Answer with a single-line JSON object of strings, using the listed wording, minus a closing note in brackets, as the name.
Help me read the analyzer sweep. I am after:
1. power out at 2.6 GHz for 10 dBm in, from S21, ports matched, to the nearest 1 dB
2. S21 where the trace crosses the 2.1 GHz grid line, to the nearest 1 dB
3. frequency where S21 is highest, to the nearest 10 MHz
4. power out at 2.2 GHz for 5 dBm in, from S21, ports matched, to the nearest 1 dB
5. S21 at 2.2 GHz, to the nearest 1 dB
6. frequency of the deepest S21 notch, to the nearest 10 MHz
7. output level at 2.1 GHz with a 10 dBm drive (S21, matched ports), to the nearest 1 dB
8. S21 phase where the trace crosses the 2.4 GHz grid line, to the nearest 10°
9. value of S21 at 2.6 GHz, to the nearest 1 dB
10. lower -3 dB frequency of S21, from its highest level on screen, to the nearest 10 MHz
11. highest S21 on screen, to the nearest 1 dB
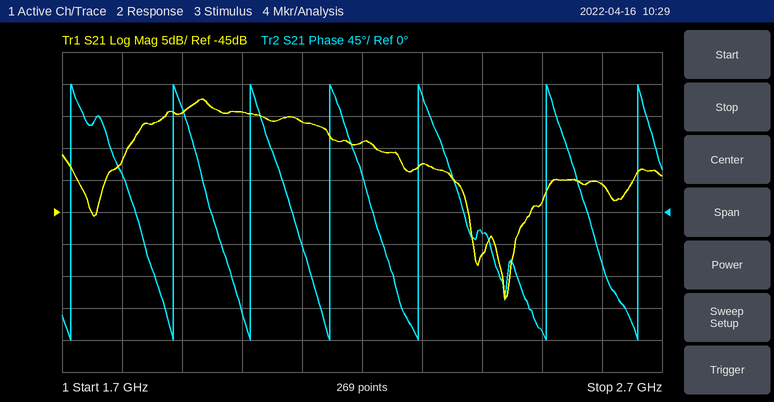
{"power out at 2.6 GHz for 10 dBm in, from S21, ports matched, to the nearest 1 dB": "-31 dBm", "S21 where the trace crosses the 2.1 GHz grid line, to the nearest 1 dB": "-31 dB", "frequency where S21 is highest, to the nearest 10 MHz": "1.93 GHz", "power out at 2.2 GHz for 5 dBm in, from S21, ports matched, to the nearest 1 dB": "-29 dBm", "S21 at 2.2 GHz, to the nearest 1 dB": "-34 dB", "frequency of the deepest S21 notch, to the nearest 10 MHz": "2.44 GHz", "output level at 2.1 GHz with a 10 dBm drive (S21, matched ports), to the nearest 1 dB": "-21 dBm", "S21 phase where the trace crosses the 2.4 GHz grid line, to the nearest 10°": "-30°", "value of S21 at 2.6 GHz, to the nearest 1 dB": "-41 dB", "lower -3 dB frequency of S21, from its highest level on screen, to the nearest 10 MHz": "1.87 GHz", "highest S21 on screen, to the nearest 1 dB": "-27 dB"}
